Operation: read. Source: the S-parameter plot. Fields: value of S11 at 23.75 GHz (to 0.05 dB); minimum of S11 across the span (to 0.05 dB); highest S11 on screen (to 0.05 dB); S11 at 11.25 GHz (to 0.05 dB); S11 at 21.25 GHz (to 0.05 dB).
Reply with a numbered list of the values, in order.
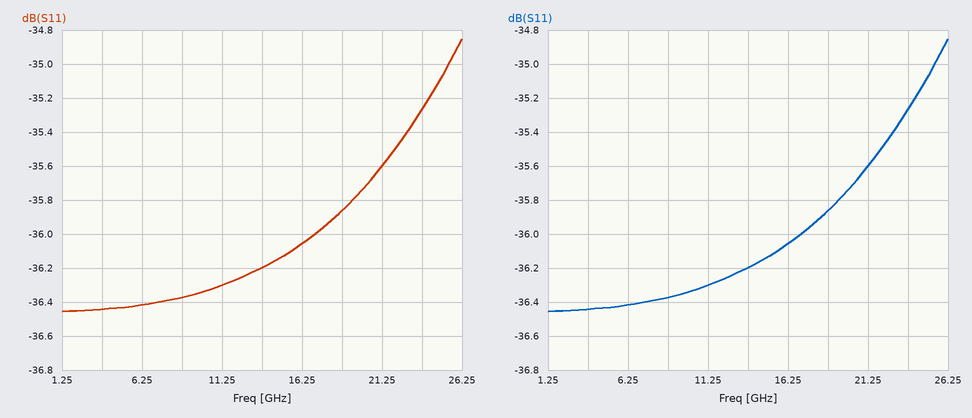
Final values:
1. -35.25 dB
2. -36.45 dB
3. -34.85 dB
4. -36.30 dB
5. -35.60 dB
